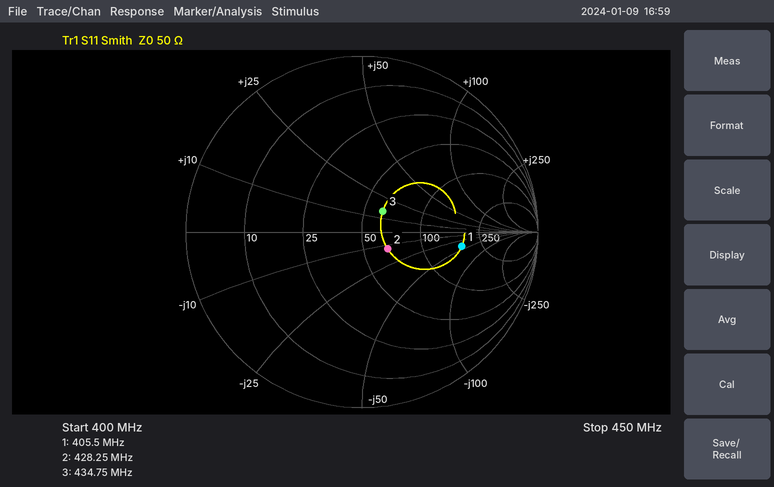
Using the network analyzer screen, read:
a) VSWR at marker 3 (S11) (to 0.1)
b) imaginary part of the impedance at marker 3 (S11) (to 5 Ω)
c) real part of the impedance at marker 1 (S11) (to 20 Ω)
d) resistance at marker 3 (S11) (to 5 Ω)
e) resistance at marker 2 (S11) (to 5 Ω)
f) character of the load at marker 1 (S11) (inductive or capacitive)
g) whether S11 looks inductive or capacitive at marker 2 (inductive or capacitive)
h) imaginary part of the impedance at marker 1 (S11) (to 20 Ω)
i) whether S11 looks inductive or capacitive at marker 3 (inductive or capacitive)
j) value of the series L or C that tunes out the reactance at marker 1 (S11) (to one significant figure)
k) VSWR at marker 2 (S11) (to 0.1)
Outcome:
1.4
+15 Ω
180 Ω
60 Ω
65 Ω
capacitive
capacitive
-40 Ω
inductive
20 nH
1.4
